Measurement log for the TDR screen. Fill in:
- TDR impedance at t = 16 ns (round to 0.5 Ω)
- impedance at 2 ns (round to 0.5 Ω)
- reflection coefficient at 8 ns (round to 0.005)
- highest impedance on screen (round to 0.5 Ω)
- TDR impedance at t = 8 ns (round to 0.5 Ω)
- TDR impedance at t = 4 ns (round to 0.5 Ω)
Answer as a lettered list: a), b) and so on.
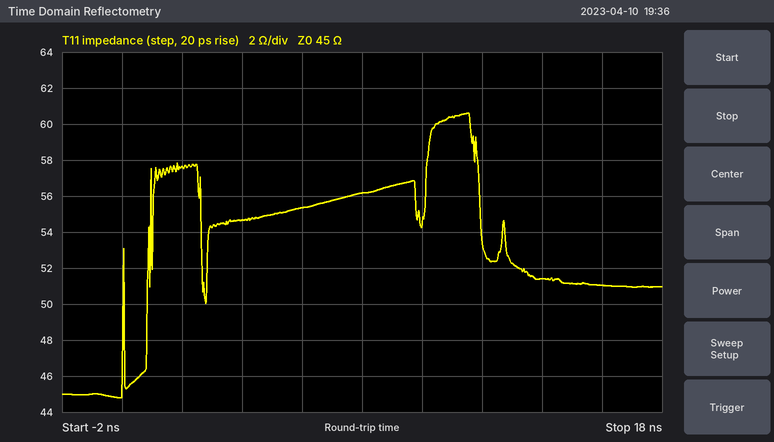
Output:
a) 51.0 Ω
b) 57.5 Ω
c) +0.110
d) 60.5 Ω
e) 56.0 Ω
f) 54.5 Ω
